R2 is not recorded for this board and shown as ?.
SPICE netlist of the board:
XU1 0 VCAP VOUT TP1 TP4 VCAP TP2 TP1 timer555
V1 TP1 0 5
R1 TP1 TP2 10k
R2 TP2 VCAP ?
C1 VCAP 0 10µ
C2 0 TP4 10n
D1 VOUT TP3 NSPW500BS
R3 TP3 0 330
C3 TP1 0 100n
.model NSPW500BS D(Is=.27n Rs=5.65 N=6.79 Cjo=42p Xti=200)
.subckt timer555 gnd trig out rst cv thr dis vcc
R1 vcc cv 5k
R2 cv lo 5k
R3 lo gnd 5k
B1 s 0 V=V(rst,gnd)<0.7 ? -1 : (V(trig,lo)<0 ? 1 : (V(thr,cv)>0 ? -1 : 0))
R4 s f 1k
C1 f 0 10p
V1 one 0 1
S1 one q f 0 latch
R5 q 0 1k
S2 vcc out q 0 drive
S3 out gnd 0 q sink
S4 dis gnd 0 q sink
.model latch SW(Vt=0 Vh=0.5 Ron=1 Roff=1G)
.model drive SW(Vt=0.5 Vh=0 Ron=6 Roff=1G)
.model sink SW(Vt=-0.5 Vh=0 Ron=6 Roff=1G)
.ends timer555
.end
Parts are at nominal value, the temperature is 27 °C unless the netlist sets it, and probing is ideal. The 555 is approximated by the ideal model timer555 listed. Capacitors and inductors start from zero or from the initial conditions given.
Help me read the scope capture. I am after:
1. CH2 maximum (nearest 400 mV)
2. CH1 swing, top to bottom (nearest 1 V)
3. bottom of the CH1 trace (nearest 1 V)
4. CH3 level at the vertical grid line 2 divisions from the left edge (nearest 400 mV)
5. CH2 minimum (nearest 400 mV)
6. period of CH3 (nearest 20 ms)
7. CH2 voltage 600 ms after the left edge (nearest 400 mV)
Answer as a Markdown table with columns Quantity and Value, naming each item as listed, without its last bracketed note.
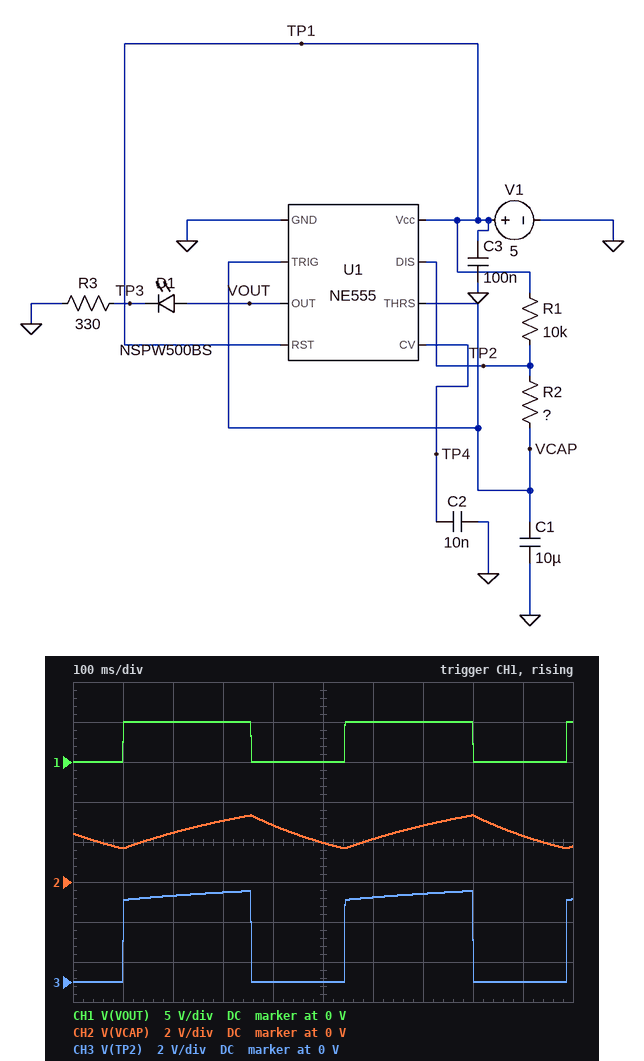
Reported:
| Quantity | Value |
|---|---|
| CH2 maximum | 3.2 V |
| CH1 swing, top to bottom | 5 V |
| bottom of the CH1 trace | 0 V |
| CH3 level at the vertical grid line 2 divisions from the left edge | 4.4 V |
| CH2 minimum | 1.6 V |
| period of CH3 | 440 ms |
| CH2 voltage 600 ms after the left edge | 2.0 V |
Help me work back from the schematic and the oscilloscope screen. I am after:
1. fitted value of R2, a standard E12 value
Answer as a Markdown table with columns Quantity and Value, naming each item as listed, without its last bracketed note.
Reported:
| Quantity | Value |
|---|---|
| fitted value of R2, a standard E12 value | 27 kΩ |
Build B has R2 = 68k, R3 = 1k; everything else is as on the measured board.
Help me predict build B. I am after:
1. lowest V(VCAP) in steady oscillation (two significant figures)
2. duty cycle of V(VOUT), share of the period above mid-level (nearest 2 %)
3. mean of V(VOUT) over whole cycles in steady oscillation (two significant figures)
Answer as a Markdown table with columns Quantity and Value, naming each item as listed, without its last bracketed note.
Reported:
| Quantity | Value |
|---|---|
| lowest V(VCAP) in steady oscillation | 1.7 V |
| duty cycle of V(VOUT), share of the period above mid-level | 54 % |
| mean of V(VOUT) over whole cycles in steady oscillation | 2.7 V |
